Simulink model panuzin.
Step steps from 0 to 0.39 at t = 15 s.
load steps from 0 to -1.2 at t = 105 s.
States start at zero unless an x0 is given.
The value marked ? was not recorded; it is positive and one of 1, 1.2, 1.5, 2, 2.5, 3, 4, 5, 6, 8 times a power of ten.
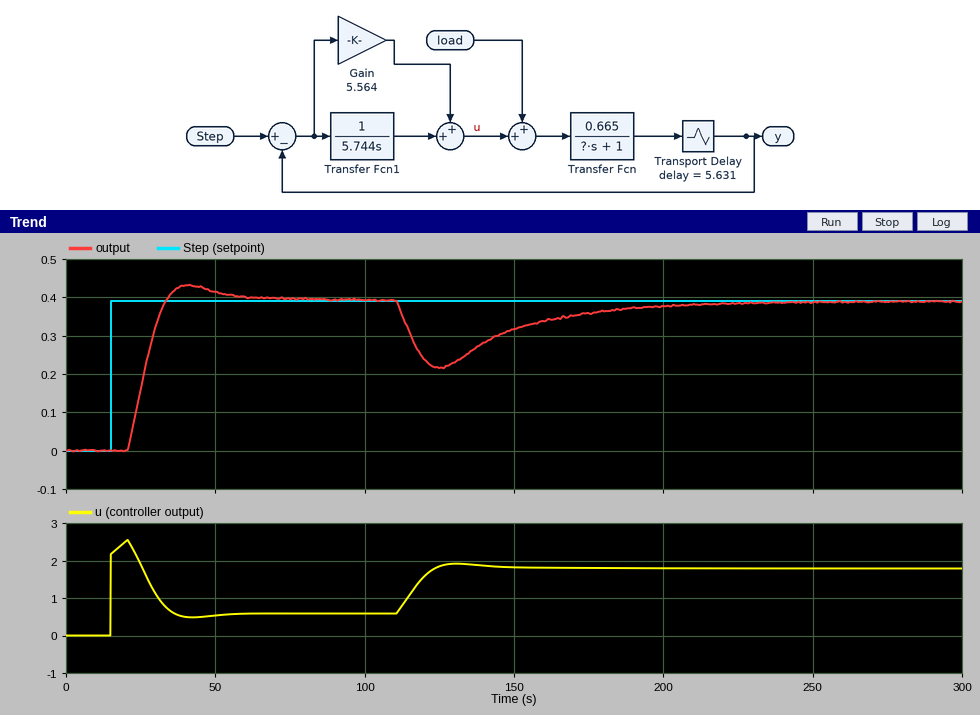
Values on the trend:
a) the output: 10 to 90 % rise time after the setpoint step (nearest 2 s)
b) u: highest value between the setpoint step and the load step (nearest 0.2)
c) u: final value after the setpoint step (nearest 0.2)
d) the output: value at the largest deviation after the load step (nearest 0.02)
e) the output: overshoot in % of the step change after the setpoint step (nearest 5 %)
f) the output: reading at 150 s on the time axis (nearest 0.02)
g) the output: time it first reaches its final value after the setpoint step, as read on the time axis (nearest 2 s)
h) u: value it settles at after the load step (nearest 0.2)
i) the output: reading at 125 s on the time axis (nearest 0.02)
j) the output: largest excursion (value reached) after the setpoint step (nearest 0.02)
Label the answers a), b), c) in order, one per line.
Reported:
a) 10 s
b) 2.6
c) 0.6
d) 0.22
e) 10 %
f) 0.32
g) 34 s
h) 1.8
i) 0.22
j) 0.44
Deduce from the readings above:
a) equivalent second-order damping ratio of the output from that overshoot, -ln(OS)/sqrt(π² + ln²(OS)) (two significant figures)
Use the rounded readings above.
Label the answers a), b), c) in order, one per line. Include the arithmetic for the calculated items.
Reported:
a) ln(0.1) = -2.303; 2.303 / sqrt(9.870 + 5.302) = 0.59
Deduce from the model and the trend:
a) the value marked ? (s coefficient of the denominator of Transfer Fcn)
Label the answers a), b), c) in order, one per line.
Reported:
a) 40
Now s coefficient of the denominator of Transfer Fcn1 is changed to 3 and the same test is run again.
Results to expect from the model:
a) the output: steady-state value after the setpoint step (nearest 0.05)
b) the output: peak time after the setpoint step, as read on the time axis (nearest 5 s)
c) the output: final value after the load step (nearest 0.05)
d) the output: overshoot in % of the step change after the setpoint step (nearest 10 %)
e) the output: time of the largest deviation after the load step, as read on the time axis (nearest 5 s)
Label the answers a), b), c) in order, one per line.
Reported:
a) 0.40
b) 40 s
c) 0.40
d) 30 %
e) 125 s
